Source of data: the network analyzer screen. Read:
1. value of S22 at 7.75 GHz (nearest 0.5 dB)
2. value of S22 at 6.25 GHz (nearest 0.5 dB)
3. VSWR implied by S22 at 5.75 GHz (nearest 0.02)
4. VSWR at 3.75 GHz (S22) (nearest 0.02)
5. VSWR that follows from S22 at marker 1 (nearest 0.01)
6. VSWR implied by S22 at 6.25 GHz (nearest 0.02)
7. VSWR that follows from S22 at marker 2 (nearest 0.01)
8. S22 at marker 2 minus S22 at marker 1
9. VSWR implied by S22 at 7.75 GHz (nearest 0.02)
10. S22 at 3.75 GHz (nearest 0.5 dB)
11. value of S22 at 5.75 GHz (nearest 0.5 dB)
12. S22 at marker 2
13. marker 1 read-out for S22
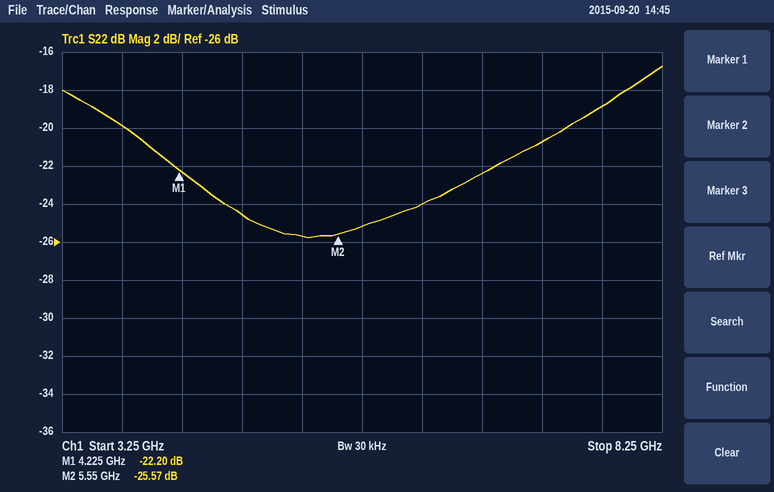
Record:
-19.0 dB
-24.0 dB
1.12
1.22
1.17
1.14
1.11
-3.37 dB
1.26
-20.0 dB
-25.0 dB
-25.57 dB
-22.20 dB
